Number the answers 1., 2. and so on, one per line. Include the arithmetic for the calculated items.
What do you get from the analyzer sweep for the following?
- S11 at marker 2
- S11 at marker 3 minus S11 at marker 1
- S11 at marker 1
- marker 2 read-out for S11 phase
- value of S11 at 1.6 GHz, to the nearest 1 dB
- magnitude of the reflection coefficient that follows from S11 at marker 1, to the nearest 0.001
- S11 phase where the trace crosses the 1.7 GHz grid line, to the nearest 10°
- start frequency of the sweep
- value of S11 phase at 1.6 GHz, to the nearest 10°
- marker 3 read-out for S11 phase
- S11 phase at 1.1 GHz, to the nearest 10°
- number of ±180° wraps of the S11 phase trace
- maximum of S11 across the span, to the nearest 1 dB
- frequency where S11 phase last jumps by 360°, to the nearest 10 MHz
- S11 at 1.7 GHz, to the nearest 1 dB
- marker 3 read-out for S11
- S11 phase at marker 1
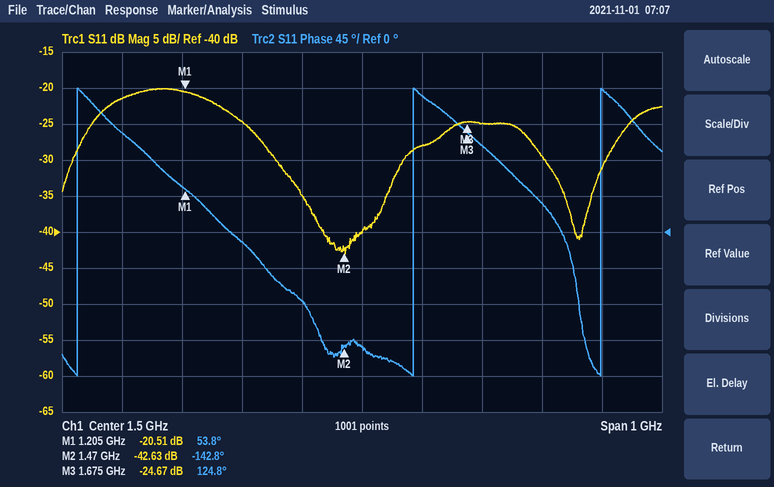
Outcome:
1. -42.63 dB
2. -24.67 − (-20.51) = -4.16 dB
3. -20.51 dB
4. -142.8°
5. -28 dB
6. 10^(-20.51/20) ≈ 0.094
7. 110°
8. 1 GHz
9. 170°
10. 124.8°
11. 120°
12. 3
13. -20 dB
14. 1.90 GHz
15. -25 dB
16. -24.67 dB
17. 53.8°
